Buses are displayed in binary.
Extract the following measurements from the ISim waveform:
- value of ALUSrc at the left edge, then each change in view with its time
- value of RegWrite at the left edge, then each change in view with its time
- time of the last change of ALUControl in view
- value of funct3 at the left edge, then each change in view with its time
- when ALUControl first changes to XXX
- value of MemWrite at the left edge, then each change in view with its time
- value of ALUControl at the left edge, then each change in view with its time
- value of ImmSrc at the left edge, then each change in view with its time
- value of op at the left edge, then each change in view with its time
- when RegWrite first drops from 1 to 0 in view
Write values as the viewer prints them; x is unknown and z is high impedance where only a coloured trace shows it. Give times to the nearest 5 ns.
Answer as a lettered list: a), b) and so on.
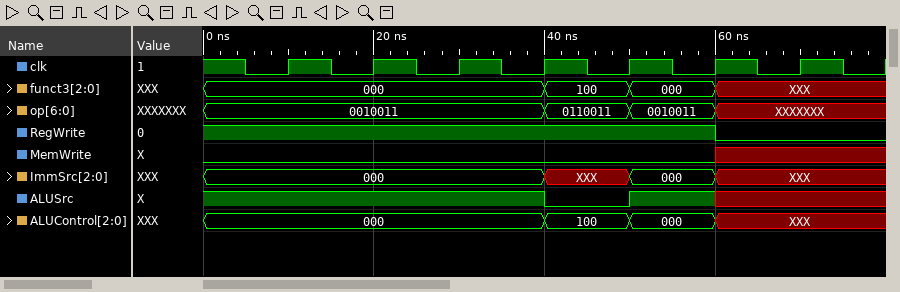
a) 1, 0 at 40 ns, 1 at 50 ns, x at 60 ns
b) 1, 0 at 60 ns
c) 60 ns
d) 000, 100 at 40 ns, 000 at 50 ns, XXX at 60 ns
e) 60 ns
f) 0, x at 60 ns
g) 000, 100 at 40 ns, 000 at 50 ns, XXX at 60 ns
h) 000, XXX at 40 ns, 000 at 50 ns, XXX at 60 ns
i) 0010011, 0110011 at 40 ns, 0010011 at 50 ns, XXXXXXX at 60 ns
j) 60 ns
